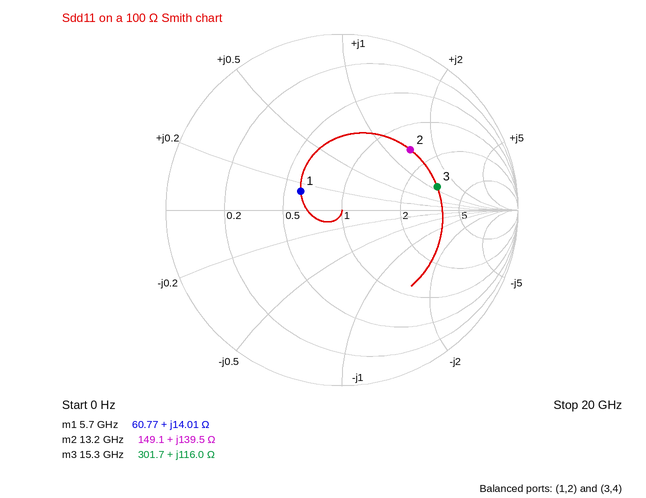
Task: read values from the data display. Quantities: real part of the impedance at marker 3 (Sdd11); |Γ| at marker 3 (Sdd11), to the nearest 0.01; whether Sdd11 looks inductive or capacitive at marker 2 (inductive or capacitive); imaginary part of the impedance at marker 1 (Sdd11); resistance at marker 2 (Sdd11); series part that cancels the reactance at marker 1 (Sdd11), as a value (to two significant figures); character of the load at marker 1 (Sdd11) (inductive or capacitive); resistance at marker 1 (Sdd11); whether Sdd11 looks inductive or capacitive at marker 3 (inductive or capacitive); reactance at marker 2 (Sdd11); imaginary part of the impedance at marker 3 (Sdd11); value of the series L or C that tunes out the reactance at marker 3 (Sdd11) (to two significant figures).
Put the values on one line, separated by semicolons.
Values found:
301.7 Ω; 0.56; inductive; +14.01 Ω; 149.1 Ω; 2.0 pF; inductive; 60.77 Ω; inductive; +139.5 Ω; +116.0 Ω; 90 fF
